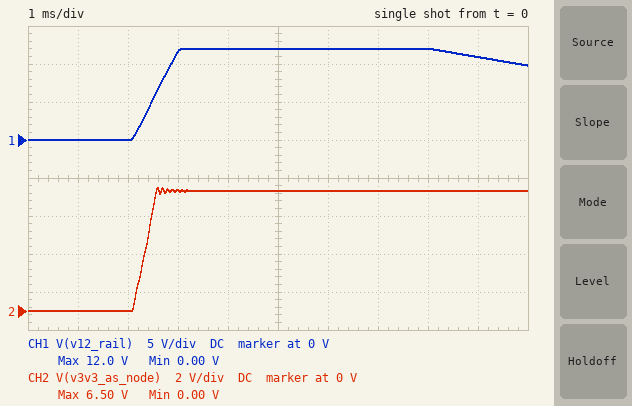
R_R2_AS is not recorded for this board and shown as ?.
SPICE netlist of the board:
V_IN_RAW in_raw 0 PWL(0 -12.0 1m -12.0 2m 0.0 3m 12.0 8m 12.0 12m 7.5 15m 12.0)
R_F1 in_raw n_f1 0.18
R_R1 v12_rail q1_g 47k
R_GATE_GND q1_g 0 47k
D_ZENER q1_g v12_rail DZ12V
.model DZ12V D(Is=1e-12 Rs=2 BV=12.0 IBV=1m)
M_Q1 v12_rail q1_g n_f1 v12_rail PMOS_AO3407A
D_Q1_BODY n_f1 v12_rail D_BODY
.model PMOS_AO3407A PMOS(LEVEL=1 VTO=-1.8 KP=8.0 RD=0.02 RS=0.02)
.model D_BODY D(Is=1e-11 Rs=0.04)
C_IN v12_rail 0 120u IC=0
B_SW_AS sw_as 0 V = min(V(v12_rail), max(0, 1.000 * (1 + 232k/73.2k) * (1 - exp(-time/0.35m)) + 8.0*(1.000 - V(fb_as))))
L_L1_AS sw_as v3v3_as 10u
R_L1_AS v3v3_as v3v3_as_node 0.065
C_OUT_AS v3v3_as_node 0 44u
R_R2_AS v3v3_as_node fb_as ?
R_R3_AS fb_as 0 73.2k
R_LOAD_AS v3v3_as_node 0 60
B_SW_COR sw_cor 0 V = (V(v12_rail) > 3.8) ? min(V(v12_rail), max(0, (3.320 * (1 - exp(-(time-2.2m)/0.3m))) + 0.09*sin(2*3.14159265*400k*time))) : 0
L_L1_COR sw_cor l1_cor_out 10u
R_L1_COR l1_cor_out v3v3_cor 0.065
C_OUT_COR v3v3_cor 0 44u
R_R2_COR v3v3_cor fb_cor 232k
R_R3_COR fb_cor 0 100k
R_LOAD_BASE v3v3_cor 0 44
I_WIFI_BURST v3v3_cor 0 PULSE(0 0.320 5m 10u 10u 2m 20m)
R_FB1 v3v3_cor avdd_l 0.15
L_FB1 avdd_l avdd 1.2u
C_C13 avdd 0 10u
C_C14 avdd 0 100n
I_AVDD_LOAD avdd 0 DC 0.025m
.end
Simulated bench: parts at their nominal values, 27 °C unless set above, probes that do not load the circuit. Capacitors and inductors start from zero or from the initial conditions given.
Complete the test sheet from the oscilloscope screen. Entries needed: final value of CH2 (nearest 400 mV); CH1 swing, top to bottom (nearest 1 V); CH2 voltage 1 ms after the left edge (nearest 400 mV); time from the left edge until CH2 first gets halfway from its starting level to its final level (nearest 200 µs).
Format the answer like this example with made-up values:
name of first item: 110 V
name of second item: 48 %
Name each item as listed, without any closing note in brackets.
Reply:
final value of CH2: 6.4 V
CH1 swing, top to bottom: 12 V
CH2 voltage 1 ms after the left edge: 0 V
time from the left edge until CH2 first gets halfway from its starting level to its final level: 2.4 ms
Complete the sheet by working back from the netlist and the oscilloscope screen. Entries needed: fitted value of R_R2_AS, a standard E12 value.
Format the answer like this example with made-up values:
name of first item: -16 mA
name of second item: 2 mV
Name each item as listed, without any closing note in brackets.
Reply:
fitted value of R_R2_AS, a standard E12 value: 560 kΩ
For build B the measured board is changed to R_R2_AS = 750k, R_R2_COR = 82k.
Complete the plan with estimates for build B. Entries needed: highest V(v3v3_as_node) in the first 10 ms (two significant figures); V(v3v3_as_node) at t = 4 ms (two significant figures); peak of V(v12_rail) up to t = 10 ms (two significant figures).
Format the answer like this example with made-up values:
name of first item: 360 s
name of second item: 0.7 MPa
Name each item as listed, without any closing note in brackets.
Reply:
highest V(v3v3_as_node) in the first 10 ms: 7.3 V
V(v3v3_as_node) at t = 4 ms: 7.1 V
peak of V(v12_rail) up to t = 10 ms: 12 V
